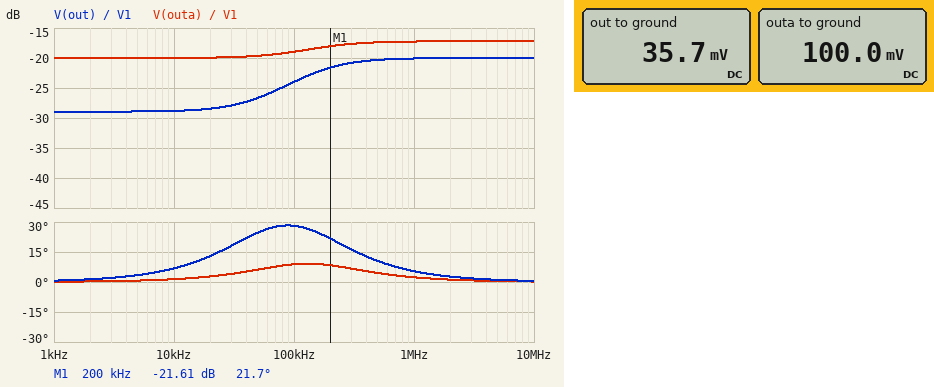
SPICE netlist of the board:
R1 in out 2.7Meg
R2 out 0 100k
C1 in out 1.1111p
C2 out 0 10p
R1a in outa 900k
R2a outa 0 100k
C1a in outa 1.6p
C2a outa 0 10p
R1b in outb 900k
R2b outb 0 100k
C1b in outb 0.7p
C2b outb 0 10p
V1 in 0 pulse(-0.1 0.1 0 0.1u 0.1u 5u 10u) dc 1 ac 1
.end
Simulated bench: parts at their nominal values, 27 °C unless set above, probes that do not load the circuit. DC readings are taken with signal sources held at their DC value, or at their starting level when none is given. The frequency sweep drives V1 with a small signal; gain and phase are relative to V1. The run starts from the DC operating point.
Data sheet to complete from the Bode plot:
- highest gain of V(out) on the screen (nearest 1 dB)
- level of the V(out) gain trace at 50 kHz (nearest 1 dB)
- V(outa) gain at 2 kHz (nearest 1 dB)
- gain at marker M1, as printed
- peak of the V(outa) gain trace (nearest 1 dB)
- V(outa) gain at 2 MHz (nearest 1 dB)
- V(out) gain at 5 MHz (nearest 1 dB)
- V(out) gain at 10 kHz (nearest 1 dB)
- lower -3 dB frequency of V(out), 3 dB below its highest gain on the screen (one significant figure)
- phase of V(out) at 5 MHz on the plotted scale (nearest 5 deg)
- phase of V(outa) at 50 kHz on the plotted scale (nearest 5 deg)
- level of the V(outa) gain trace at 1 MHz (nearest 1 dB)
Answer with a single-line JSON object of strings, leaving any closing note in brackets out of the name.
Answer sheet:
{"highest gain of V(out) on the screen": "-20 dB", "level of the V(out) gain trace at 50 kHz": "-27 dB", "V(outa) gain at 2 kHz": "-20 dB", "gain at marker M1, as printed": "-21.61 dB", "peak of the V(outa) gain trace": "-17 dB", "V(outa) gain at 2 MHz": "-17 dB", "V(out) gain at 5 MHz": "-20 dB", "V(out) gain at 10 kHz": "-29 dB", "lower -3 dB frequency of V(out), 3 dB below its highest gain on the screen": "100 kHz", "phase of V(out) at 5 MHz on the plotted scale": "0 deg", "phase of V(outa) at 50 kHz on the plotted scale": "5 deg", "level of the V(outa) gain trace at 1 MHz": "-17 dB"}
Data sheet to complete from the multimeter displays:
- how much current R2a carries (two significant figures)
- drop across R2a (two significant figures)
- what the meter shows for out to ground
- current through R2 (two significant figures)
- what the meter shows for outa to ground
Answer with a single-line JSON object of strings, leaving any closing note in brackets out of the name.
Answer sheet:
{"how much current R2a carries": "1.0 µA", "drop across R2a": "100 mV", "what the meter shows for out to ground": "35.7 mV", "current through R2": "360 nA", "what the meter shows for outa to ground": "100.0 mV"}
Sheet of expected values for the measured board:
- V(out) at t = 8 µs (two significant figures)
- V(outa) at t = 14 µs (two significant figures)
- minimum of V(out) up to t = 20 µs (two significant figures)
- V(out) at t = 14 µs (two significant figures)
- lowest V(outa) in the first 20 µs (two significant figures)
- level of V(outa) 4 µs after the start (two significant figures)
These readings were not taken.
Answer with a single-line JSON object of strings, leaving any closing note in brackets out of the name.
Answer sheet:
{"V(out) at t = 8 µs": "-4.5 mV", "V(outa) at t = 14 µs": "10 mV", "minimum of V(out) up to t = 20 µs": "-16 mV", "V(out) at t = 14 µs": "3.9 mV", "lowest V(outa) in the first 20 µs": "-17 mV", "level of V(outa) 4 µs after the start": "10 mV"}
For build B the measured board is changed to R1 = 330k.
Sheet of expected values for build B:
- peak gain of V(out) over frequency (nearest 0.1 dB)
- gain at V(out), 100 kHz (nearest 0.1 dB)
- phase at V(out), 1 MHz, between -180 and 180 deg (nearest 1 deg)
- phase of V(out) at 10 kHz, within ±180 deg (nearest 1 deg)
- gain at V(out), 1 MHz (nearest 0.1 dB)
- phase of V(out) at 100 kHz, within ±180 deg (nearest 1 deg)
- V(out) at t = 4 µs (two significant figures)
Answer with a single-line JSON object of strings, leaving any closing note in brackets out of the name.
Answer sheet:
{"peak gain of V(out) over frequency": "-12.7 dB", "gain at V(out), 100 kHz": "-13.5 dB", "phase at V(out), 1 MHz, between -180 and 180 deg": "-13 deg", "phase of V(out) at 10 kHz, within ±180 deg": "-2 deg", "gain at V(out), 1 MHz": "-19.4 dB", "phase of V(out) at 100 kHz, within ±180 deg": "-15 deg", "V(out) at t = 4 µs": "23 mV"}
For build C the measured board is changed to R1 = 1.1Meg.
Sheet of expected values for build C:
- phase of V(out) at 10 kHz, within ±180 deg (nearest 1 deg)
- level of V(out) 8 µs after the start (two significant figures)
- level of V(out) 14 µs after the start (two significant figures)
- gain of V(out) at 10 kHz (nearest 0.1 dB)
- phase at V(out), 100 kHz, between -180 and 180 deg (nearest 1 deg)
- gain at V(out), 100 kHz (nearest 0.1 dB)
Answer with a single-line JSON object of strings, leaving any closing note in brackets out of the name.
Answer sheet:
{"phase of V(out) at 10 kHz, within ±180 deg": "1 deg", "level of V(out) 8 µs after the start": "-8.5 mV", "level of V(out) 14 µs after the start": "8.4 mV", "gain of V(out) at 10 kHz": "-21.6 dB", "phase at V(out), 100 kHz, between -180 and 180 deg": "5 deg", "gain at V(out), 100 kHz": "-21.1 dB"}
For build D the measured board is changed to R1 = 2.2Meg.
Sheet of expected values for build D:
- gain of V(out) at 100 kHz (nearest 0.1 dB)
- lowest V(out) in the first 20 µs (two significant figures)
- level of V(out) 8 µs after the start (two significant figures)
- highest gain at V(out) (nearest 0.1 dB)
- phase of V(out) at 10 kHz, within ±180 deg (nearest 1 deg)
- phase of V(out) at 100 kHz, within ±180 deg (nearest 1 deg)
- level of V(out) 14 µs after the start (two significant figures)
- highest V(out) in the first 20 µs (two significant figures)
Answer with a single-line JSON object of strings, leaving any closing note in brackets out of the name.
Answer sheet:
{"gain of V(out) at 100 kHz": "-23.6 dB", "lowest V(out) in the first 20 µs": "-15 mV", "level of V(out) 8 µs after the start": "-5.1 mV", "highest gain at V(out)": "-20.0 dB", "phase of V(out) at 10 kHz, within ±180 deg": "5 deg", "phase of V(out) at 100 kHz, within ±180 deg": "23 deg", "level of V(out) 14 µs after the start": "4.6 mV", "highest V(out) in the first 20 µs": "15 mV"}
